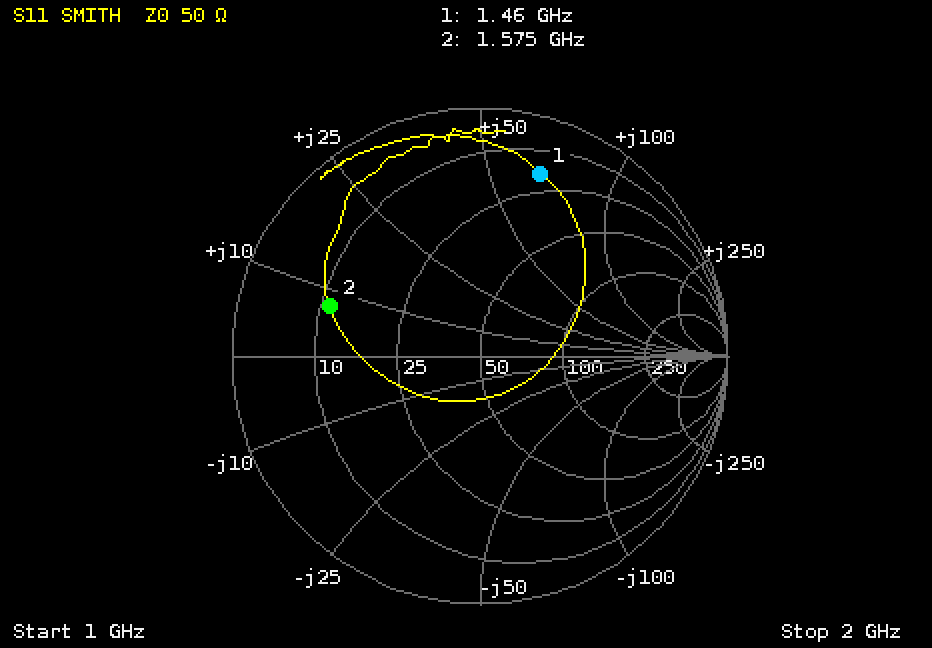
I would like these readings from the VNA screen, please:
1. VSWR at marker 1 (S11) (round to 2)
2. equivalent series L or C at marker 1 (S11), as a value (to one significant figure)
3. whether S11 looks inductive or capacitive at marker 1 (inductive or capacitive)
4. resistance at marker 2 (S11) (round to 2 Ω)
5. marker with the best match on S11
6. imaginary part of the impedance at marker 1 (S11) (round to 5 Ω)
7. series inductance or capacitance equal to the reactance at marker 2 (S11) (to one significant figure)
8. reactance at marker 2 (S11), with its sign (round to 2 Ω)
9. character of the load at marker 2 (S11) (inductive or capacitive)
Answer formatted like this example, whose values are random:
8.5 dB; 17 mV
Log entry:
8; 7 nH; inductive; 12 Ω; marker 2; +65 Ω; 800 pH; +8 Ω; inductive
